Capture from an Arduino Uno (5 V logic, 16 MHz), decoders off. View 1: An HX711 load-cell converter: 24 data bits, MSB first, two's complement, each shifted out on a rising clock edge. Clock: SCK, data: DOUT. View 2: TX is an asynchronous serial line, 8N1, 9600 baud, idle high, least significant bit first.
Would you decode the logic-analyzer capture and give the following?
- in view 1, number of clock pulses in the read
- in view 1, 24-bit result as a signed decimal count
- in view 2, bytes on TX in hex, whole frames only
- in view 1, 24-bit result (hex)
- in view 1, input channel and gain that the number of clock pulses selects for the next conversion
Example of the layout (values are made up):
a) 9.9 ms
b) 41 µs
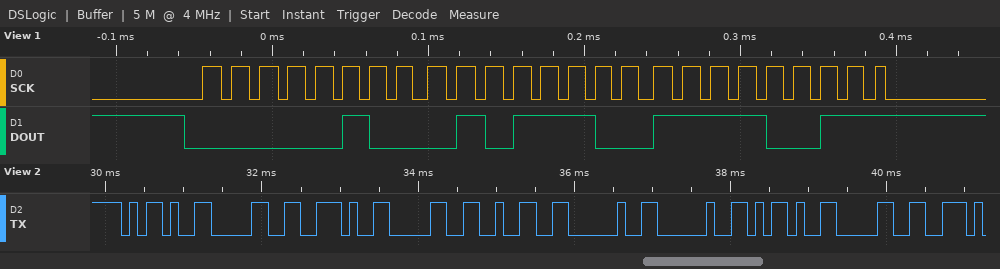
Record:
a) 25
b) 285939
c) 2D 30 2E 30 32 20 20 2D 30
d) 0x045CF3
e) channel A, gain 128
